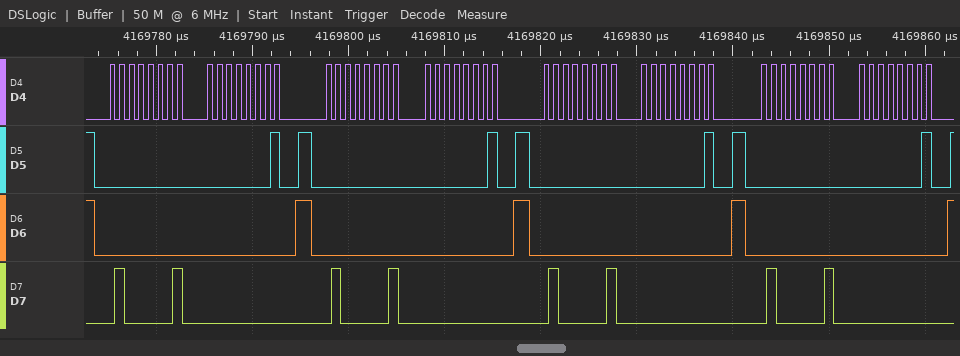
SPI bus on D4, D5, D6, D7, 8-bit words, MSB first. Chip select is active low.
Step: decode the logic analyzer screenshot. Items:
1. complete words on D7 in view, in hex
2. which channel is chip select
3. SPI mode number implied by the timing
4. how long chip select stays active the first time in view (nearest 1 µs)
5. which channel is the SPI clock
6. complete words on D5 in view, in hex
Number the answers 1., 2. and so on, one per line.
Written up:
1. 41, 00, 41, 00, 41, 00, 41, 00
2. D6
3. 0
4. 21 µs
5. D4
6. 00, 01, 00, 01, 00, 01, 00, 01
